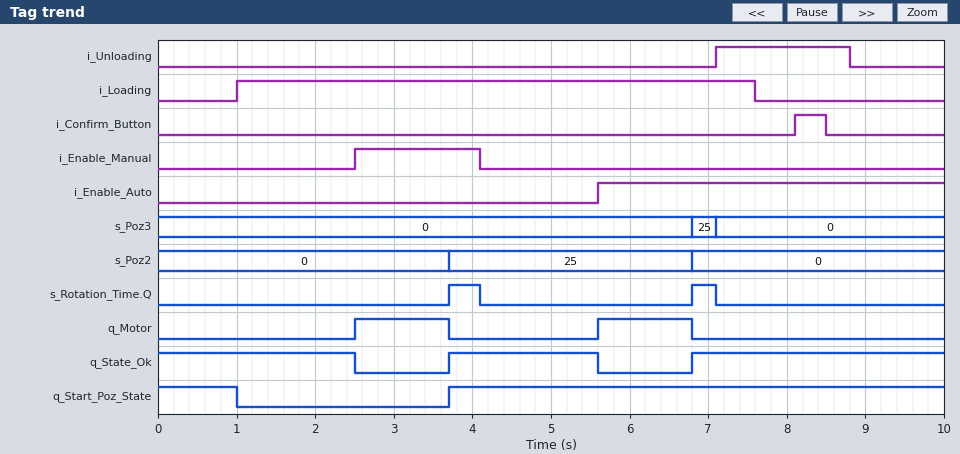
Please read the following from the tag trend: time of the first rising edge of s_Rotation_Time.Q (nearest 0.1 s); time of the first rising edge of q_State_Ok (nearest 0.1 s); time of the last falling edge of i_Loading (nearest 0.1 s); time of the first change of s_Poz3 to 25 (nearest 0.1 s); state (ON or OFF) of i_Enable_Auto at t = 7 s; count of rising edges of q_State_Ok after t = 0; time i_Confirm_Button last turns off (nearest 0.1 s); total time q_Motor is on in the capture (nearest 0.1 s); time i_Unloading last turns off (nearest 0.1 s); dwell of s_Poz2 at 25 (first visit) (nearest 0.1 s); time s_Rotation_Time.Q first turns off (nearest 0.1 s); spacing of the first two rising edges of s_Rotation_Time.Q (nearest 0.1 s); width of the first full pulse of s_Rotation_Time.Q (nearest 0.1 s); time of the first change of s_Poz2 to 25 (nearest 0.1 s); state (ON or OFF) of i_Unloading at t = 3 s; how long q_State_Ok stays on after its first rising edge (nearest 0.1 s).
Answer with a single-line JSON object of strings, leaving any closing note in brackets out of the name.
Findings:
{"time of the first rising edge of s_Rotation_Time.Q": "3.7 s", "time of the first rising edge of q_State_Ok": "3.7 s", "time of the last falling edge of i_Loading": "7.6 s", "time of the first change of s_Poz3 to 25": "6.8 s", "state (ON or OFF) of i_Enable_Auto at t = 7 s": "ON", "count of rising edges of q_State_Ok after t = 0": "2", "time i_Confirm_Button last turns off": "8.5 s", "total time q_Motor is on in the capture": "2.4 s", "time i_Unloading last turns off": "8.8 s", "dwell of s_Poz2 at 25 (first visit)": "3.1 s", "time s_Rotation_Time.Q first turns off": "4.1 s", "spacing of the first two rising edges of s_Rotation_Time.Q": "3.1 s", "width of the first full pulse of s_Rotation_Time.Q": "0.4 s", "time of the first change of s_Poz2 to 25": "3.7 s", "state (ON or OFF) of i_Unloading at t = 3 s": "OFF", "how long q_State_Ok stays on after its first rising edge": "1.9 s"}
